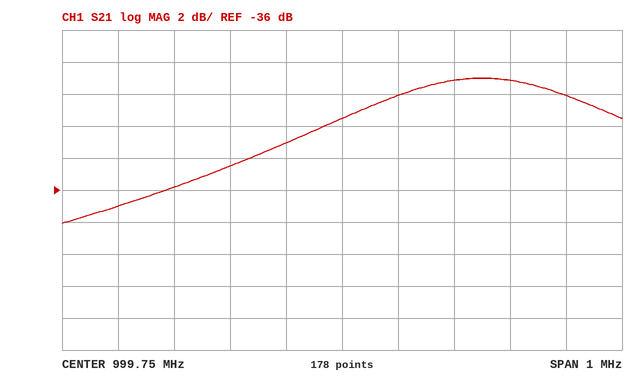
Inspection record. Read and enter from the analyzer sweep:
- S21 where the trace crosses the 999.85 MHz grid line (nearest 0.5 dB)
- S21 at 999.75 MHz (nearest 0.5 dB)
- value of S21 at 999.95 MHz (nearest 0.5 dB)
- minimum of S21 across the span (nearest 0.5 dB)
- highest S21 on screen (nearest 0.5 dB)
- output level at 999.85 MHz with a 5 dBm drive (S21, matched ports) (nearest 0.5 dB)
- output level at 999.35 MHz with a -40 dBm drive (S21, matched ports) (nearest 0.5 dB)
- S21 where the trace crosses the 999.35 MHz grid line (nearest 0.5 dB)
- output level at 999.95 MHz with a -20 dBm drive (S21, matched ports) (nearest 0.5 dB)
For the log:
-30.0 dB
-31.5 dB
-29.0 dB
-38.0 dB
-29.0 dB
-25.0 dBm
-77.0 dBm
-37.0 dB
-49.0 dBm
